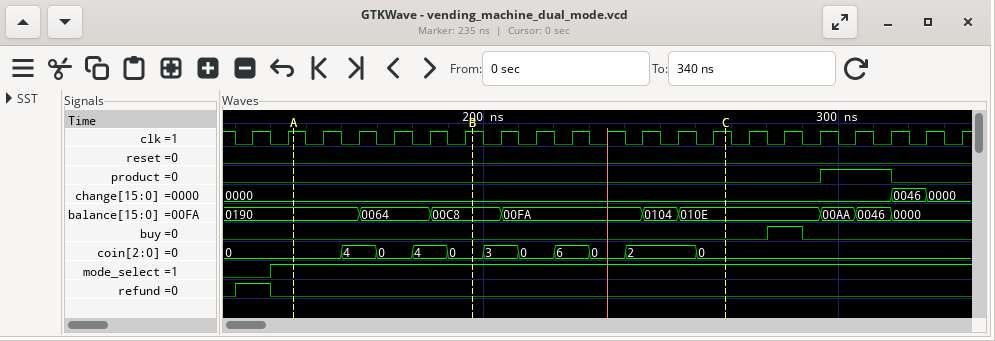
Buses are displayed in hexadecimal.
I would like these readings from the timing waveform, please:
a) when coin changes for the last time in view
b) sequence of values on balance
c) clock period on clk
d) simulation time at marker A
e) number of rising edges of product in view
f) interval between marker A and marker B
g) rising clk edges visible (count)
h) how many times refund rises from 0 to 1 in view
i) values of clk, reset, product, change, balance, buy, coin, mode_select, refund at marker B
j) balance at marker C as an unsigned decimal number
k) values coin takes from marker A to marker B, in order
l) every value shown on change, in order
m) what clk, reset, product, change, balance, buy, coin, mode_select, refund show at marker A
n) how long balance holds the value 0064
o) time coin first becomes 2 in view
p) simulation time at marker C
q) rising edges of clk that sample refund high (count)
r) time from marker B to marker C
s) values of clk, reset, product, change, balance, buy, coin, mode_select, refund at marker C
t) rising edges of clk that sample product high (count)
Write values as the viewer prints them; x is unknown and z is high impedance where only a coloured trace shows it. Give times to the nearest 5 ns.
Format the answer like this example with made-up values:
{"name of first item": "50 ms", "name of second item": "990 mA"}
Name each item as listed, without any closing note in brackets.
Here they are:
{"when coin changes for the last time in view": "260 ns", "sequence of values on balance": "0190, 0064, 00C8, 00FA, 0104, 010E, 00AA, 0046, 0000", "clock period on clk": "10 ns", "simulation time at marker A": "145 ns", "number of rising edges of product in view": "1", "interval between marker A and marker B": "50 ns", "rising clk edges visible": "21", "how many times refund rises from 0 to 1 in view": "1", "values of clk, reset, product, change, balance, buy, coin, mode_select, refund at marker B": "clk=1, reset=0, product=0, change=0000, balance=00C8, buy=0, coin=0, mode_select=1, refund=0", "balance at marker C as an unsigned decimal number": "270", "values coin takes from marker A to marker B, in order": "0, 4, 0, 4, 0", "every value shown on change, in order": "0000, 0046, 0000", "what clk, reset, product, change, balance, buy, coin, mode_select, refund show at marker A": "clk=1, reset=0, product=0, change=0000, balance=0190, buy=0, coin=0, mode_select=1, refund=0", "how long balance holds the value 0064": "20 ns", "time coin first becomes 2 in view": "240 ns", "simulation time at marker C": "270 ns", "rising edges of clk that sample refund high": "1", "time from marker B to marker C": "70 ns", "values of clk, reset, product, change, balance, buy, coin, mode_select, refund at marker C": "clk=1, reset=0, product=0, change=0000, balance=010E, buy=0, coin=0, mode_select=1, refund=0", "rising edges of clk that sample product high": "2"}
